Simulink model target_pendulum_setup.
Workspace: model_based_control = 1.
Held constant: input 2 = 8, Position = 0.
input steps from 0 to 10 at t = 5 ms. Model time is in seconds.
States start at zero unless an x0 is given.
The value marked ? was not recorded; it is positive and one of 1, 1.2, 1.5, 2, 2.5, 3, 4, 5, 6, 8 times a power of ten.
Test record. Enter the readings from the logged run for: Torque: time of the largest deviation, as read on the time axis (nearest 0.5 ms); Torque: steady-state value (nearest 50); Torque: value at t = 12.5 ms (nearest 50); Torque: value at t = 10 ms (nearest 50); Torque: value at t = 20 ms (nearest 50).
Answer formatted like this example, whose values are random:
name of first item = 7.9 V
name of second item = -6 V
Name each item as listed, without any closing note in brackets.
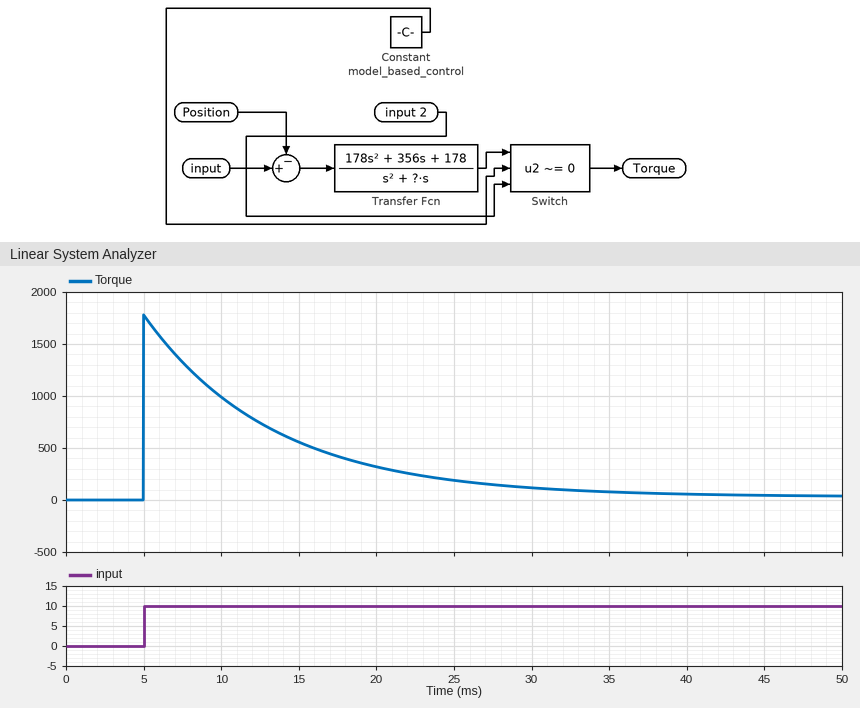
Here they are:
Torque: time of the largest deviation, as read on the time axis = 5.0 ms
Torque: steady-state value = 50
Torque: value at t = 12.5 ms = 750
Torque: value at t = 10 ms = 1000
Torque: value at t = 20 ms = 300
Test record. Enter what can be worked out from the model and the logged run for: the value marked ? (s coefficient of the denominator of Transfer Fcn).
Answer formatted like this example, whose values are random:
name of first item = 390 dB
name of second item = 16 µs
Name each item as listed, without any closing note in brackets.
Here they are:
the value marked ? = 120
